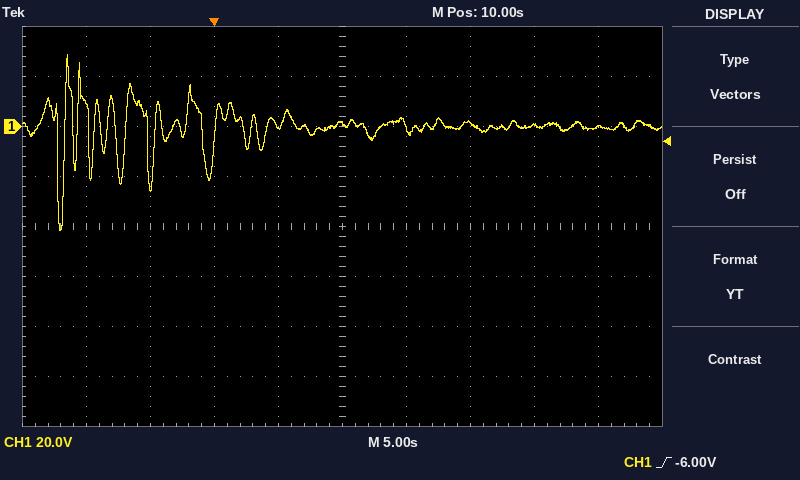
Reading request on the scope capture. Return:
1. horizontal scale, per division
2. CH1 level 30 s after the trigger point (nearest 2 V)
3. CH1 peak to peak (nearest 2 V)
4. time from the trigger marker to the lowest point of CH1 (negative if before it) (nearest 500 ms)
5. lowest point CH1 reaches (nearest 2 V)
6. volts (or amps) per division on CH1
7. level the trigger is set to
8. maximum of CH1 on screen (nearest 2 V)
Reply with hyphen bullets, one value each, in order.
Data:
- 5 s
- 0 V
- 70 V
- -12.0 s
- -42 V
- 20 V
- -6.00 V
- 28 V
